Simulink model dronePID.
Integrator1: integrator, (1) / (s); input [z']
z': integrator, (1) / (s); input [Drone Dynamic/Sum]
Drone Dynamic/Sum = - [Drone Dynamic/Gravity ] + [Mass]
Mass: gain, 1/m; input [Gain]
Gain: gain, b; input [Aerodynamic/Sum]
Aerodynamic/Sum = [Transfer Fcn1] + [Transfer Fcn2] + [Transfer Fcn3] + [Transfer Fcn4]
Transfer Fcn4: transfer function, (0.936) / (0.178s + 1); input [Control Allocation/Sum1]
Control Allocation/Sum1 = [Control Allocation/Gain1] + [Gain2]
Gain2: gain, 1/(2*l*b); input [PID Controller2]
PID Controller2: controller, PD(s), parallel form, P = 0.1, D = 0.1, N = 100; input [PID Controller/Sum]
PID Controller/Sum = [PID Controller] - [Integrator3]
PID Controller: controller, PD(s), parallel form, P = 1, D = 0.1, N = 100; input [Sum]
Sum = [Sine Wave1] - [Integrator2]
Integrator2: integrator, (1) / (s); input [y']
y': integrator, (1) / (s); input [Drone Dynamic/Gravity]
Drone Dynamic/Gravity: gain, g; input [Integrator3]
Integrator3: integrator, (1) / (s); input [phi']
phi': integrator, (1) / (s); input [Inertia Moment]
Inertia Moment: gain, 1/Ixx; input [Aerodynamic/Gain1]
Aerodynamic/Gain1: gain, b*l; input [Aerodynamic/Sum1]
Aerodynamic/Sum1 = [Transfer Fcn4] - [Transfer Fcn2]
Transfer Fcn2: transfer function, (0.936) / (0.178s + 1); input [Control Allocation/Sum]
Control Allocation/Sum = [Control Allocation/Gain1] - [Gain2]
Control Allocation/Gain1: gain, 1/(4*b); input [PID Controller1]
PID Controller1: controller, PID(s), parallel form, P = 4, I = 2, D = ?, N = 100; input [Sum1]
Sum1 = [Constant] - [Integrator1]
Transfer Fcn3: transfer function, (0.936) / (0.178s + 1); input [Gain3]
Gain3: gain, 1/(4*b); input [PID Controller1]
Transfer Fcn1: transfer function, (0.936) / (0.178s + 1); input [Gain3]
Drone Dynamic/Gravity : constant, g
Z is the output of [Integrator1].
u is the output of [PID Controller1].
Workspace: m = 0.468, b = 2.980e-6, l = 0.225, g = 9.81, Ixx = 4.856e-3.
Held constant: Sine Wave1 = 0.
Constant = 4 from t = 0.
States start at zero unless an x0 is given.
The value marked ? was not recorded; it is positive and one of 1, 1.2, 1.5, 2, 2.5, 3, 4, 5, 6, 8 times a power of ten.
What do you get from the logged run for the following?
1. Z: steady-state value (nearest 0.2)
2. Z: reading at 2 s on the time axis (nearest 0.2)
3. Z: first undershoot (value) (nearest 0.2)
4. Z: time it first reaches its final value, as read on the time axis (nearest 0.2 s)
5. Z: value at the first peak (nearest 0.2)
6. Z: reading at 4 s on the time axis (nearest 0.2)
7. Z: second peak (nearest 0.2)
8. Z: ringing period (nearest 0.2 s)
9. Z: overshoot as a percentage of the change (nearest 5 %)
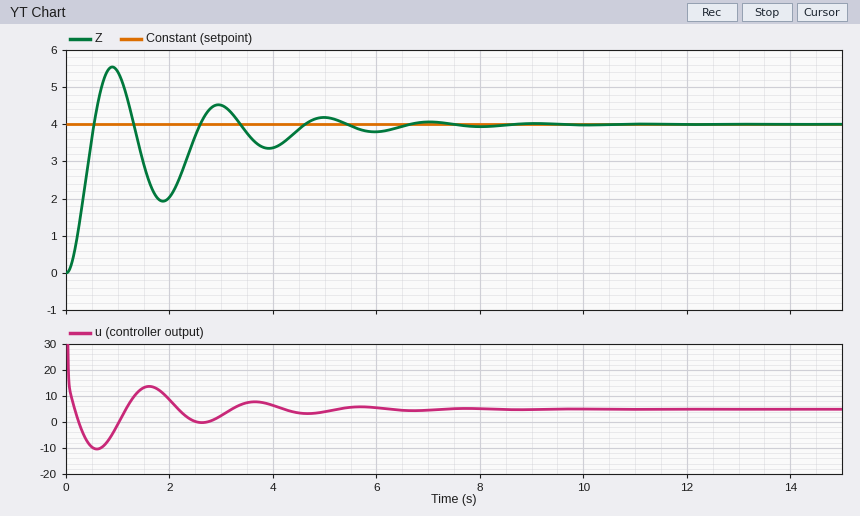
4.0
2.0
2.0
0.6 s
5.6
3.4
4.6
2.0 s
40 %
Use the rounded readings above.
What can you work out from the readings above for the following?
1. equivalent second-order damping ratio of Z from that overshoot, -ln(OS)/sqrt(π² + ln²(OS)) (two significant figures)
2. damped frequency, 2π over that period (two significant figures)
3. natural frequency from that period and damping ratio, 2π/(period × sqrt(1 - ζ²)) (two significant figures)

0.28
3.1 rad/s
3.3 rad/s
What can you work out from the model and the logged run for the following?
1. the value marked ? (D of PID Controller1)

1.5
